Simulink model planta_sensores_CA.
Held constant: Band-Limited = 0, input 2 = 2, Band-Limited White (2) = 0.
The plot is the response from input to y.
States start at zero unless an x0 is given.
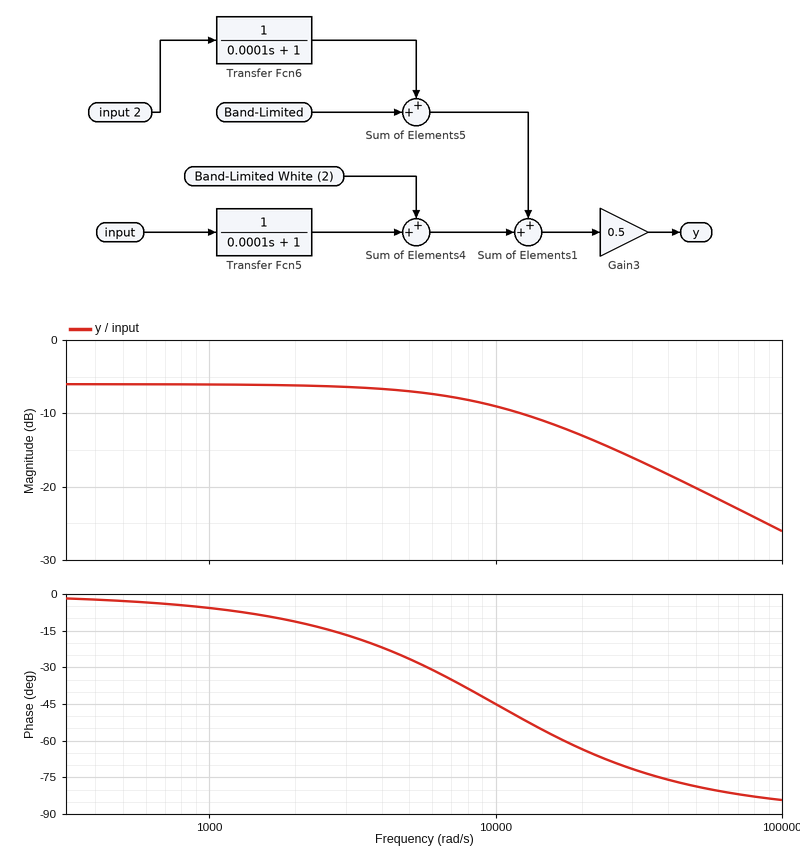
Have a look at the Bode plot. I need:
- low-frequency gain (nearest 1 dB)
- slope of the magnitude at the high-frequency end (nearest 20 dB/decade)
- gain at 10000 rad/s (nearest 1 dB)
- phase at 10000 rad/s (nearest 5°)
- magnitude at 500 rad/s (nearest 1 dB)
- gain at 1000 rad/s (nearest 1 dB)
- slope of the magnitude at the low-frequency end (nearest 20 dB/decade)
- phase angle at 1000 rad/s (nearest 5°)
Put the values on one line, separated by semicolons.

-6 dB; -20 dB/decade; -9 dB; -45°; -6 dB; -6 dB; 0 dB/decade; -5°
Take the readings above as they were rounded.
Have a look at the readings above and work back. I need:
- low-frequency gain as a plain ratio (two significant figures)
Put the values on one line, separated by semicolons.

0.50
